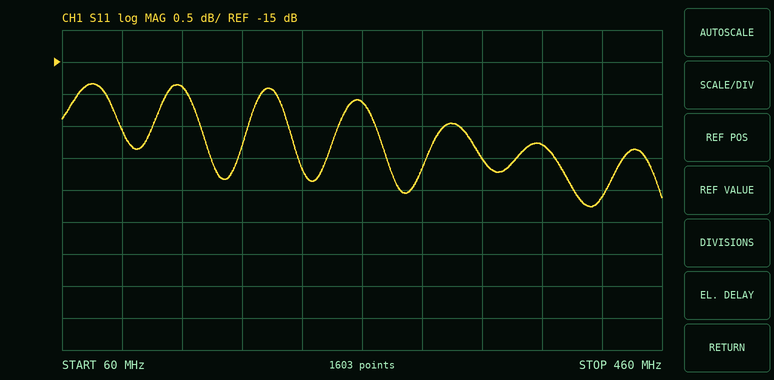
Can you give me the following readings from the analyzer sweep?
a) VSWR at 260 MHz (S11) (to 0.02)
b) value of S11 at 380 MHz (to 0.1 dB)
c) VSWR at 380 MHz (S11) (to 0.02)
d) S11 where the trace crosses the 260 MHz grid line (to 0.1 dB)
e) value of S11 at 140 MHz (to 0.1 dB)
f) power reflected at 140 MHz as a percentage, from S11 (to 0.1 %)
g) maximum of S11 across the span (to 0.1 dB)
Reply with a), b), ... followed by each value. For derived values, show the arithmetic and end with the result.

a) |Γ| = 10^(-15.6/20) = 0.1660; VSWR = (1 + 0.1660)/(1 − 0.1660) ≈ 1.40
b) -16.3 dB
c) |Γ| = 10^(-16.3/20) = 0.1531; VSWR = (1 + 0.1531)/(1 − 0.1531) ≈ 1.36
d) -15.6 dB
e) -15.4 dB
f) 10^(-15.4/10) ≈ 2.9 %
g) -15.3 dB
